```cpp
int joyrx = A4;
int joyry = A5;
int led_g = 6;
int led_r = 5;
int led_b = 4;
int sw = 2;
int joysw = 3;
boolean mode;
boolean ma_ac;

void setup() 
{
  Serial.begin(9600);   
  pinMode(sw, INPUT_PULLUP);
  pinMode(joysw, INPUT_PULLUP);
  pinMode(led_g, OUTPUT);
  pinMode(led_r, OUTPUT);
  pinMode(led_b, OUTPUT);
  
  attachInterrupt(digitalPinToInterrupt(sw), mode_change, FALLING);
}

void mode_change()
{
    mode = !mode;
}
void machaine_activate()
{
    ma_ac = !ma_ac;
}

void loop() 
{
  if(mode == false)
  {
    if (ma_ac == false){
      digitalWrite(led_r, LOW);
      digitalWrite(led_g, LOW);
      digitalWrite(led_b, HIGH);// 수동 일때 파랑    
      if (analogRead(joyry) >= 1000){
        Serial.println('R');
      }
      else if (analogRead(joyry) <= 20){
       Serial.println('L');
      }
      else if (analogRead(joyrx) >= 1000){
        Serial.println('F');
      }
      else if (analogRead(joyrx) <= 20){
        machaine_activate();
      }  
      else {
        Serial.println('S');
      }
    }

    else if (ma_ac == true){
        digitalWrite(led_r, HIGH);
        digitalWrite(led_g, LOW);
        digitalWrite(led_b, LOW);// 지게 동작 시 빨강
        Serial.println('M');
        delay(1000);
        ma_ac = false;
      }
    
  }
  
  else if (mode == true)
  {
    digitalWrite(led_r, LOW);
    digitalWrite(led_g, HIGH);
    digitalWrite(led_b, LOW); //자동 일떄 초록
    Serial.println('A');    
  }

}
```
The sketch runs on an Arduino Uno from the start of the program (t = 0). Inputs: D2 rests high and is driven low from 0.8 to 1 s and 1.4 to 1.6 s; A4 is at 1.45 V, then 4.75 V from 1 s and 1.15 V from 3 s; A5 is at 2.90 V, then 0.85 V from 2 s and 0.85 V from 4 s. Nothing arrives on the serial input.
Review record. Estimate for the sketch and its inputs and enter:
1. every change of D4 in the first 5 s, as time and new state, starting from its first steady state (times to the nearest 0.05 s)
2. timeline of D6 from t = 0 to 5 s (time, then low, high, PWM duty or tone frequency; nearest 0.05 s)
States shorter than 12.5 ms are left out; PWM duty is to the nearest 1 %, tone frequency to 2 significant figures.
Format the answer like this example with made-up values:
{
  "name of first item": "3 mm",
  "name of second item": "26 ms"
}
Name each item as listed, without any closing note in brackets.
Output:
{
  "every change of D4 in the first 5 s, as time and new state, starting from its first steady state": "0 s high; 0.8 s low; 1.4 s high",
  "timeline of D6 from t = 0 to 5 s": "0 s low; 0.8 s high; 1.4 s low"
}
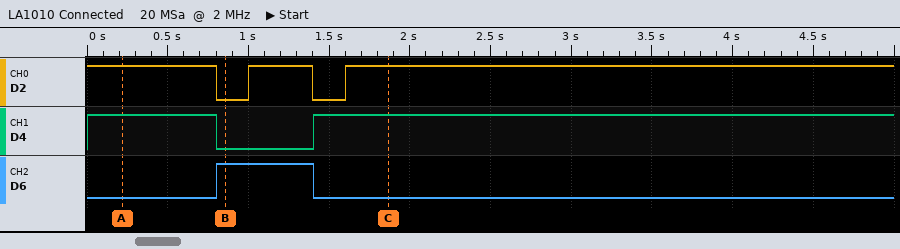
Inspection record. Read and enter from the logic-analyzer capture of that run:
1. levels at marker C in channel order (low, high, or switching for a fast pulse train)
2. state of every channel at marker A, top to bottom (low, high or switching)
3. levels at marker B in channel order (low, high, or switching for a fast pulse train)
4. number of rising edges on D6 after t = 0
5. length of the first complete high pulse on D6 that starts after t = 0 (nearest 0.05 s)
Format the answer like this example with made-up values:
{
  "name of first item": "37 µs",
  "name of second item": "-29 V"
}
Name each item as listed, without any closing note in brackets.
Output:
{
  "levels at marker C in channel order": "D2 high, D4 high, D6 low",
  "state of every channel at marker A, top to bottom": "D2 high, D4 high, D6 low",
  "levels at marker B in channel order": "D2 low, D4 low, D6 high",
  "number of rising edges on D6 after t = 0": "1",
  "length of the first complete high pulse on D6 that starts after t = 0": "0.60 s"
}
